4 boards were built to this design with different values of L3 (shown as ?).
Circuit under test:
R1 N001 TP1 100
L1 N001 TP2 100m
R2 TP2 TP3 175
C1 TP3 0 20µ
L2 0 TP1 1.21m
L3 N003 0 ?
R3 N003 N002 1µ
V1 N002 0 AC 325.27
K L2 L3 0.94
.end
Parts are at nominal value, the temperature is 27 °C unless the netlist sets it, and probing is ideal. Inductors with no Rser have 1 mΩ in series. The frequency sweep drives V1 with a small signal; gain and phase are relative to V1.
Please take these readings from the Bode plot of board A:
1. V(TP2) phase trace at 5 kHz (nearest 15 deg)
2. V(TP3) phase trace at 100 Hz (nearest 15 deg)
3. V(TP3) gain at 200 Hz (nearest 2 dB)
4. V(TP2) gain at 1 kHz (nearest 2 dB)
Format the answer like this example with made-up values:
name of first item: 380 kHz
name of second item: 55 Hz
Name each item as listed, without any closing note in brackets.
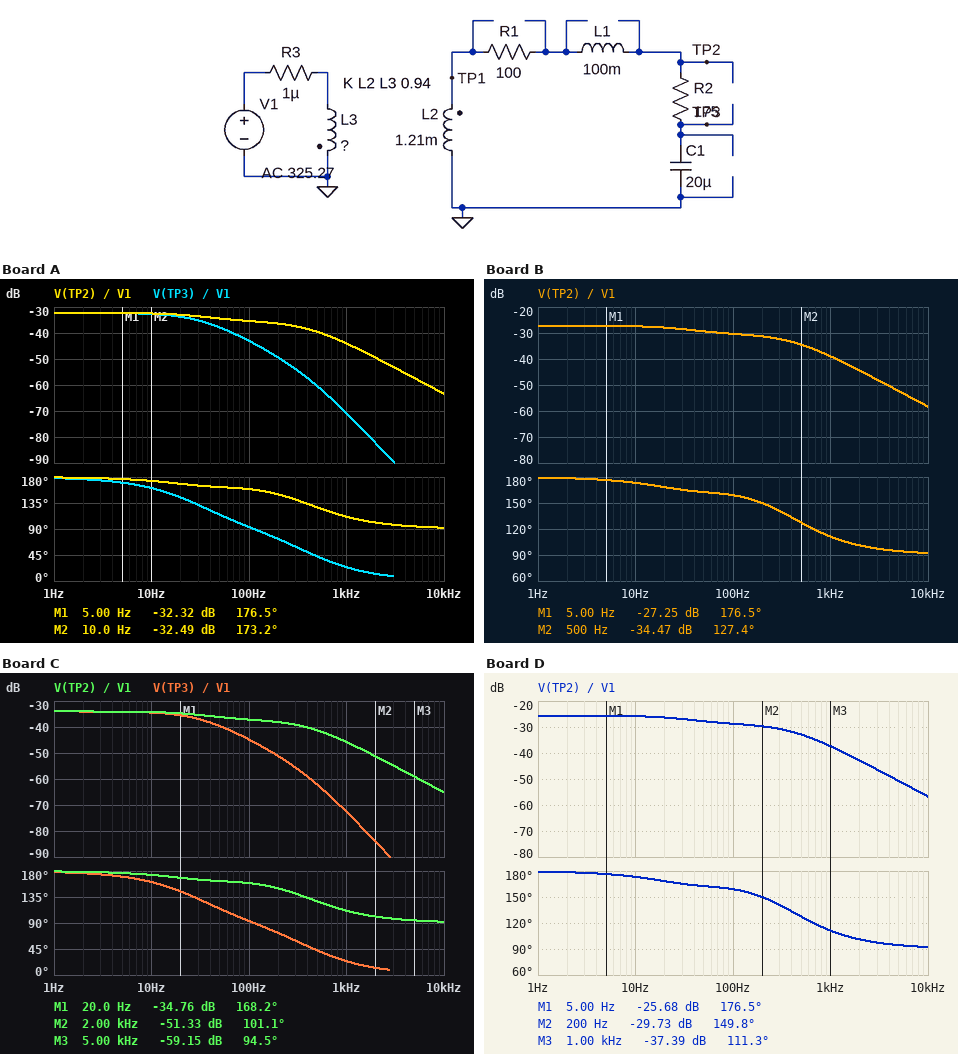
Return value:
V(TP2) phase trace at 5 kHz: 90 deg
V(TP3) phase trace at 100 Hz: 90 deg
V(TP3) gain at 200 Hz: -50 dB
V(TP2) gain at 1 kHz: -44 dB
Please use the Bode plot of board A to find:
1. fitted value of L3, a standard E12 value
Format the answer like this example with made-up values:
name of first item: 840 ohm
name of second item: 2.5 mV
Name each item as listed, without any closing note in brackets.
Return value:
fitted value of L3, a standard E12 value: 1.8 H
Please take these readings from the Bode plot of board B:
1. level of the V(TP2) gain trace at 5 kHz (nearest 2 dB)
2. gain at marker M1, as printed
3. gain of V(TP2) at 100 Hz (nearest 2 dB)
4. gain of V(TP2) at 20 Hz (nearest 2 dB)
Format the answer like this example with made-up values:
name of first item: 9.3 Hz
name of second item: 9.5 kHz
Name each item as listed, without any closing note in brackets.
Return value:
level of the V(TP2) gain trace at 5 kHz: -52 dB
gain at marker M1, as printed: -27.25 dB
gain of V(TP2) at 100 Hz: -30 dB
gain of V(TP2) at 20 Hz: -28 dB
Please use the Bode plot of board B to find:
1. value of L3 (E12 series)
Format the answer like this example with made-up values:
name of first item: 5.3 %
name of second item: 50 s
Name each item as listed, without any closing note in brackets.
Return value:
value of L3: 560 mH
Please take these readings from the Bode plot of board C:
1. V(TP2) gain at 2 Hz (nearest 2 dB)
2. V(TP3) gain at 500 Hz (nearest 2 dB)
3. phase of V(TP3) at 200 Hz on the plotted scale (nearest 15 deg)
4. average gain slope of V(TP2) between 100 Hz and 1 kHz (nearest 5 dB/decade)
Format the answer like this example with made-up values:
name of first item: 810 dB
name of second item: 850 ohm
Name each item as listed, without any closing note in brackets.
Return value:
V(TP2) gain at 2 Hz: -34 dB
V(TP3) gain at 500 Hz: -62 dB
phase of V(TP3) at 200 Hz on the plotted scale: 75 deg
average gain slope of V(TP2) between 100 Hz and 1 kHz: -10 dB/decade
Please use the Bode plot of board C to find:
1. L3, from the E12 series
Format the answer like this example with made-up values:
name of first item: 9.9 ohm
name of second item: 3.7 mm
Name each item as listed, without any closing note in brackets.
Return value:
L3, from the E12 series: 2.7 H
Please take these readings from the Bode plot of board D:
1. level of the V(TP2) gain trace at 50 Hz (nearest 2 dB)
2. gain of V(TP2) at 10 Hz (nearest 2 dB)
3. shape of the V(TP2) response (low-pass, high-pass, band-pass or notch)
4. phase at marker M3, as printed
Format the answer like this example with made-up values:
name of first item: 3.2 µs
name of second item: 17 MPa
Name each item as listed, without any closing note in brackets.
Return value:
level of the V(TP2) gain trace at 50 Hz: -28 dB
gain of V(TP2) at 10 Hz: -26 dB
shape of the V(TP2) response: low-pass
phase at marker M3, as printed: 111.3 deg
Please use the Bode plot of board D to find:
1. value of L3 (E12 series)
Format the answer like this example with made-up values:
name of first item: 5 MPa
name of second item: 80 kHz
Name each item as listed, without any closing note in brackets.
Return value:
value of L3: 390 mH
